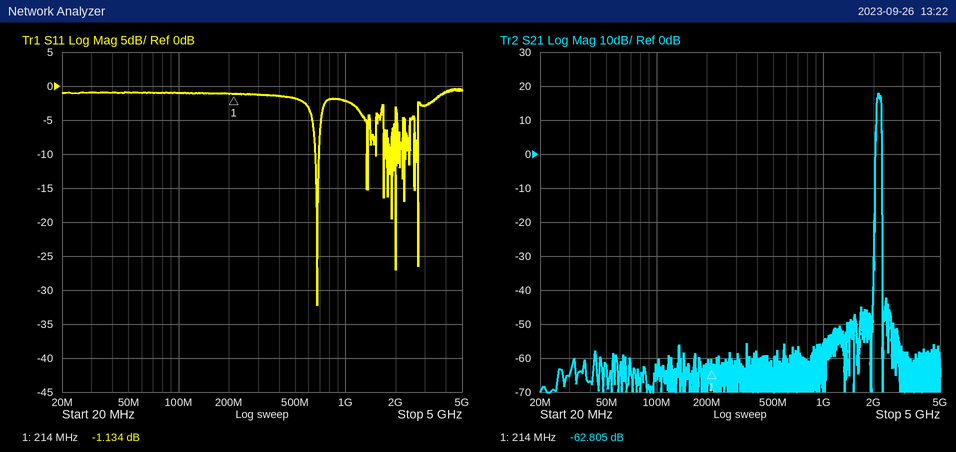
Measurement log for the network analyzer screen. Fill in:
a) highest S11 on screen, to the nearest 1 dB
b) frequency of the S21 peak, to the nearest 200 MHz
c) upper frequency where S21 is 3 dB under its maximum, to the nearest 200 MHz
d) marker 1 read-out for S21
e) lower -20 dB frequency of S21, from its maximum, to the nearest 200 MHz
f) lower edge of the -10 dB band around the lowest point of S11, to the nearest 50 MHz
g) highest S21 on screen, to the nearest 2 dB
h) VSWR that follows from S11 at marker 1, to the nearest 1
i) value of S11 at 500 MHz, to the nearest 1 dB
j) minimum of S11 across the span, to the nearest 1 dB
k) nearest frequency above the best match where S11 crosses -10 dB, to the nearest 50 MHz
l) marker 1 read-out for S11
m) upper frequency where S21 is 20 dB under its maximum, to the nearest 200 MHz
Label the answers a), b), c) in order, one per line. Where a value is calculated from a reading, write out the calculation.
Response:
a) 0 dB
b) 2.2 GHz
c) 2.2 GHz
d) -62.805 dB
e) 2.0 GHz
f) 650 MHz
g) 18 dB
h) (1 + 0.8776)/(1 − 0.8776) ≈ 15
i) -2 dB
j) -32 dB
k) 700 MHz
l) -1.134 dB
m) 2.2 GHz
